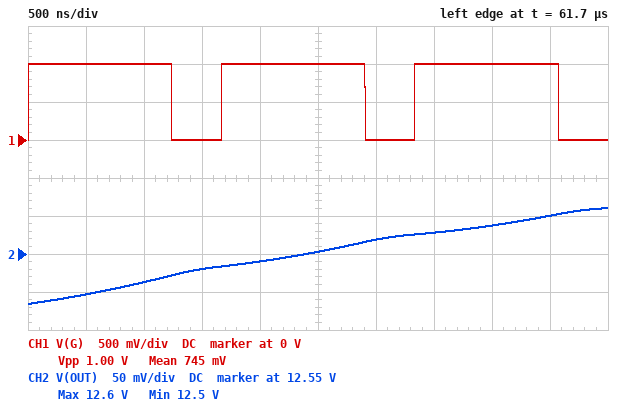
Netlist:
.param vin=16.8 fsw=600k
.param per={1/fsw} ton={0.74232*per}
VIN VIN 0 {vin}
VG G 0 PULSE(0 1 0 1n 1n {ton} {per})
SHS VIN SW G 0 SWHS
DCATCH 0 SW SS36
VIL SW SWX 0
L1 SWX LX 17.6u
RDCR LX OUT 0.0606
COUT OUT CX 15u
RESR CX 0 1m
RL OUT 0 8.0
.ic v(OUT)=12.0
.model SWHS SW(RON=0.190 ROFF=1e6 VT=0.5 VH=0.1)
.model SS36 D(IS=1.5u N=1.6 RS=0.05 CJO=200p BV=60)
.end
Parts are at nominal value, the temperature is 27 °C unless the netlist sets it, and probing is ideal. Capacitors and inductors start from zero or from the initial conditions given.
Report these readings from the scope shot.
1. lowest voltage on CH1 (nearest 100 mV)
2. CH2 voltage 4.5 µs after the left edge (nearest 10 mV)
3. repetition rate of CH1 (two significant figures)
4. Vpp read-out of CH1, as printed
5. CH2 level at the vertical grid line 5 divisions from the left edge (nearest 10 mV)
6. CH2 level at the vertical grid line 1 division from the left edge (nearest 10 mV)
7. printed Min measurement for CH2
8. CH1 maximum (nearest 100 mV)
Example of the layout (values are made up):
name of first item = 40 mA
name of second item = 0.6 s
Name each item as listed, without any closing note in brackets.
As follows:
lowest voltage on CH1 = 0 V
CH2 voltage 4.5 µs after the left edge = 12.60 V
repetition rate of CH1 = 600 kHz
Vpp read-out of CH1, as printed = 1.00 V
CH2 level at the vertical grid line 5 divisions from the left edge = 12.55 V
CH2 level at the vertical grid line 1 division from the left edge = 12.50 V
printed Min measurement for CH2 = 12.5 V
CH1 maximum = 1.0 V
